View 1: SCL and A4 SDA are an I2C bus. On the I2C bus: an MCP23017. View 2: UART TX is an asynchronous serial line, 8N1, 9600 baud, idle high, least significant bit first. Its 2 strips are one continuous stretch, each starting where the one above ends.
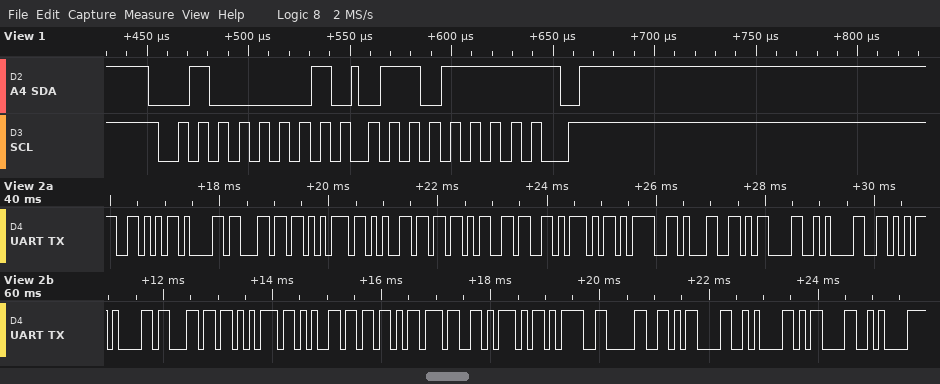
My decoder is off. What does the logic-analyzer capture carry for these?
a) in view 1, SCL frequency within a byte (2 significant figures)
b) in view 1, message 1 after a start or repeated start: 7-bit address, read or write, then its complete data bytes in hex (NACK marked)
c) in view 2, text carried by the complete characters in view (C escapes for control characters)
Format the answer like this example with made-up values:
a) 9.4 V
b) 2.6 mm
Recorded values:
a) 100 kHz
b) 0x20 read: 6F NACK
c) "Value[6]=1\r\nValue[7]=0\r\n\r\n"
